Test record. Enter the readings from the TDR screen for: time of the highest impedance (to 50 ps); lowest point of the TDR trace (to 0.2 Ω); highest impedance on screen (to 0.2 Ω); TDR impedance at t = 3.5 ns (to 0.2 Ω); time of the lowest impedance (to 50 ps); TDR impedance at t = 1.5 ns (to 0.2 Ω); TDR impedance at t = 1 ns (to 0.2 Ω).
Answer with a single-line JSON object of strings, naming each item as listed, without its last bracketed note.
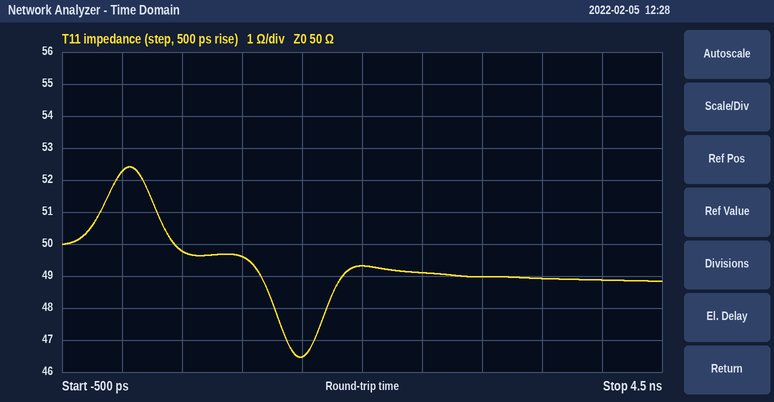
{"time of the highest impedance": "50 ps", "lowest point of the TDR trace": "46.4 Ω", "highest impedance on screen": "52.4 Ω", "TDR impedance at t = 3.5 ns": "49.0 Ω", "time of the lowest impedance": "1.50 ns", "TDR impedance at t = 1.5 ns": "46.4 Ω", "TDR impedance at t = 1 ns": "49.6 Ω"}
